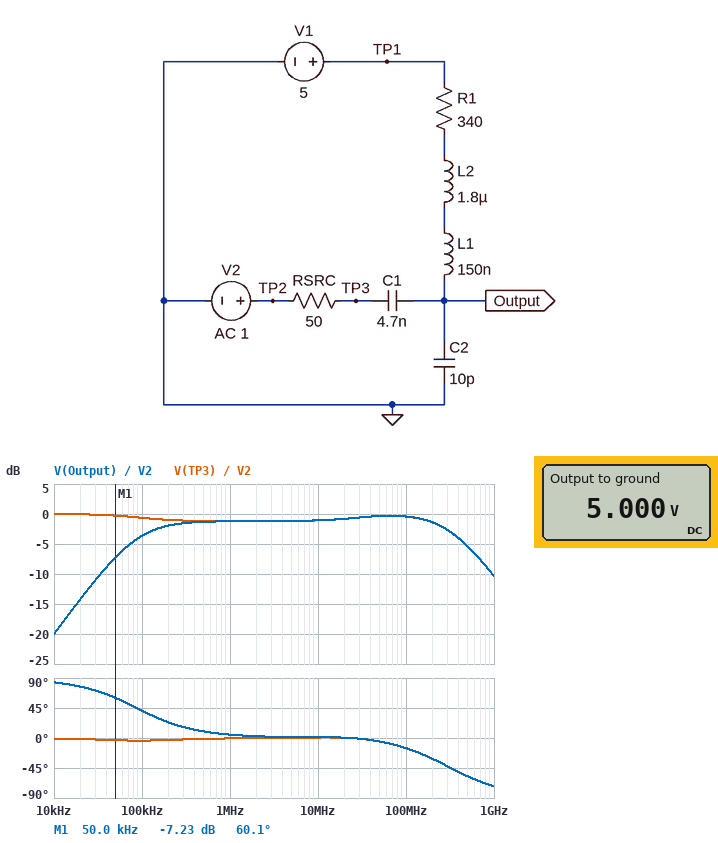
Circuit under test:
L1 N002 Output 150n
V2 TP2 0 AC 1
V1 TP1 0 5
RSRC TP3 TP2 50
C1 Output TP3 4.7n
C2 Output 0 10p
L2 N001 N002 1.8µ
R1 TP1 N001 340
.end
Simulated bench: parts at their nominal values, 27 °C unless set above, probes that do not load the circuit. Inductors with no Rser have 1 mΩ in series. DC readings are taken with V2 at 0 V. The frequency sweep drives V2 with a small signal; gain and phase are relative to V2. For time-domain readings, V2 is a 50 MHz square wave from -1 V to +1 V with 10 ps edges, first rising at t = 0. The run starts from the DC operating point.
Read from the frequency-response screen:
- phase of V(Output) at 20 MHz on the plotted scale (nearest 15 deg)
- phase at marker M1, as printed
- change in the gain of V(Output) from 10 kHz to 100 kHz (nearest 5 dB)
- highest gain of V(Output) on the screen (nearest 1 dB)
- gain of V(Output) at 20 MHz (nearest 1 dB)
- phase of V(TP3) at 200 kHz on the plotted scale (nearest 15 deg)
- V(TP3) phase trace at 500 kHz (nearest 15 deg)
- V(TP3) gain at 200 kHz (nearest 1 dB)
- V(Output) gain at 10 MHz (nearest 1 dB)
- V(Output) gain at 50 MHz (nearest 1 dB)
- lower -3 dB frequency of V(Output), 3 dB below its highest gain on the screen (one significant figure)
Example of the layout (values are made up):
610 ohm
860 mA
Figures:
0 deg
60.1 deg
15 dB
0 dB
-1 dB
0 deg
0 deg
-1 dB
-1 dB
0 dB
100 kHz
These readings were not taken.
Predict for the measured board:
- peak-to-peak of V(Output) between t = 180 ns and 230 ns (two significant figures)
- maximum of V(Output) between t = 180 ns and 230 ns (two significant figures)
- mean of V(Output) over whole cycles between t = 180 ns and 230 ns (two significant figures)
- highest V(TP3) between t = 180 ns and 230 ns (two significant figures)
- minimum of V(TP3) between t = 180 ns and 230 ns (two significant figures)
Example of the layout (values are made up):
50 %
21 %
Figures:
2.1 V
6.8 V
5.8 V
910 mV
-1.1 V
